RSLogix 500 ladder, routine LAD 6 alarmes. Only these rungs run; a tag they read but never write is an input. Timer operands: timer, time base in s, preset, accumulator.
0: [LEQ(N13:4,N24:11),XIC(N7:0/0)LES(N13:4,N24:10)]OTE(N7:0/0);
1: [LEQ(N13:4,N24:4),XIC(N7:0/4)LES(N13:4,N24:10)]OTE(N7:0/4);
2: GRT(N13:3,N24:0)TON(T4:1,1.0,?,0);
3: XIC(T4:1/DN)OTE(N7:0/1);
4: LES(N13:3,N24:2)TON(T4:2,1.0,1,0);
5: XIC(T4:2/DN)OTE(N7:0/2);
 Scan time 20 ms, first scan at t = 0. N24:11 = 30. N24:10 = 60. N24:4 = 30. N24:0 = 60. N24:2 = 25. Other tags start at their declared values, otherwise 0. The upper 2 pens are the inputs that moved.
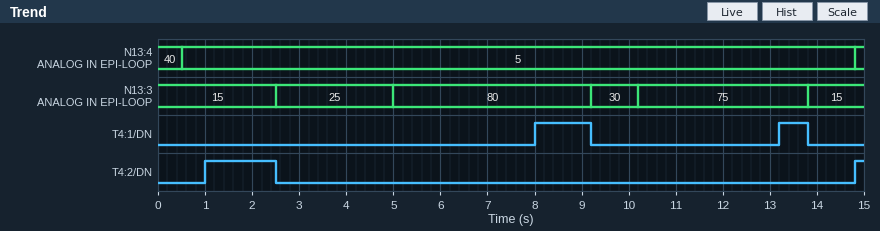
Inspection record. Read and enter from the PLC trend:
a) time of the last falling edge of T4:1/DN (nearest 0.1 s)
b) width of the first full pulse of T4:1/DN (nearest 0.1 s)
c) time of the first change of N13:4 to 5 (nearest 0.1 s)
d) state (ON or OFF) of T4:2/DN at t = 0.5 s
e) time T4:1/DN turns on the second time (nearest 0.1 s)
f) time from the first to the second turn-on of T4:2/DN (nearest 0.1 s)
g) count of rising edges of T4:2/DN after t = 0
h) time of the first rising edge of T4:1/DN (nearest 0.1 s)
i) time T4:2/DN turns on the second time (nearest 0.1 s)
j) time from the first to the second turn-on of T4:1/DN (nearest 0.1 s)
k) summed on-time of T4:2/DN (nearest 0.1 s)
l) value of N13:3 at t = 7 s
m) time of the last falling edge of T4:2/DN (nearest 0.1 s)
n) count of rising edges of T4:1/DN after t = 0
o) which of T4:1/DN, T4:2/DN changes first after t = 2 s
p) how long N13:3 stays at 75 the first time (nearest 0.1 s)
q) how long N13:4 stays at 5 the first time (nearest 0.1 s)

13.8 s
1.2 s
0.5 s
OFF
13.2 s
13.8 s
2
8.0 s
14.8 s
5.2 s
1.7 s
80
2.5 s
2
T4:2/DN
3.6 s
14.3 s
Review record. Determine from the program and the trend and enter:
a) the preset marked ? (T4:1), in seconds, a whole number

3 s
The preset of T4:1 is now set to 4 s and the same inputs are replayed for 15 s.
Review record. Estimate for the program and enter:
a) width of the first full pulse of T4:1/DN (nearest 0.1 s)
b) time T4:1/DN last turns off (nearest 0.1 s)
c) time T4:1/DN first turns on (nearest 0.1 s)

0.2 s
9.2 s
9.0 s
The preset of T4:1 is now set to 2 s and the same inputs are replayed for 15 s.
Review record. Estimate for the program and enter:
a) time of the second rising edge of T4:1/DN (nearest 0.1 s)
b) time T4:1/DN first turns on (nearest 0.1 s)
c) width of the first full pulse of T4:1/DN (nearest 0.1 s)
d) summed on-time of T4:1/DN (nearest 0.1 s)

12.2 s
7.0 s
2.2 s
3.8 s
